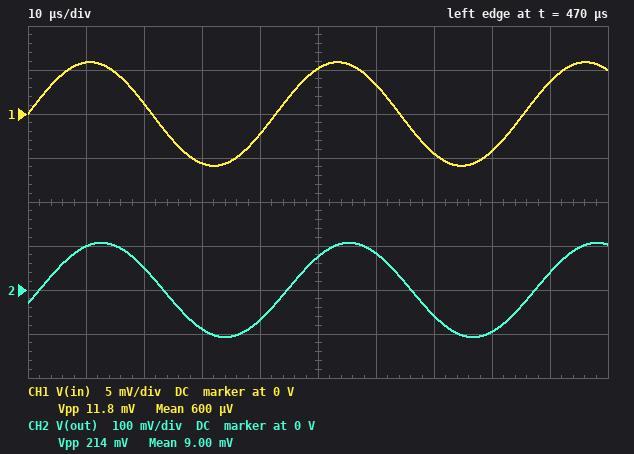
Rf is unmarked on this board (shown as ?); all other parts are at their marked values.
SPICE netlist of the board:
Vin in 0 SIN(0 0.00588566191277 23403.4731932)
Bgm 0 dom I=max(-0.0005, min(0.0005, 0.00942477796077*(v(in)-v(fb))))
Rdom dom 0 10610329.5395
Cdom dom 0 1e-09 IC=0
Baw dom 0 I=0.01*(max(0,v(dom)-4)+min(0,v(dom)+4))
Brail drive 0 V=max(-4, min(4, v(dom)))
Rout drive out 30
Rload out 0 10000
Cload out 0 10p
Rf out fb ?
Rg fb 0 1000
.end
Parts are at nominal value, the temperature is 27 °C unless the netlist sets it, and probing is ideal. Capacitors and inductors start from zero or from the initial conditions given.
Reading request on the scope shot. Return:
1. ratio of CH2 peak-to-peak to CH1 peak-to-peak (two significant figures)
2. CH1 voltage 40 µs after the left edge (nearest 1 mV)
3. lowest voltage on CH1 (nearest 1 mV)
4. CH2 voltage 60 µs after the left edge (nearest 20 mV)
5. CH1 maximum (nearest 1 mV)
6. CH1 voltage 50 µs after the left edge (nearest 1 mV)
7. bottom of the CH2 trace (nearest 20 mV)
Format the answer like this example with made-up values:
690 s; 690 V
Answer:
18; -2 mV; -6 mV; 80 mV; 6 mV; 5 mV; -100 mV
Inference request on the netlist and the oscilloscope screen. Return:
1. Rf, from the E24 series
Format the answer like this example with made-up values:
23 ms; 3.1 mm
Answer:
18 kΩ
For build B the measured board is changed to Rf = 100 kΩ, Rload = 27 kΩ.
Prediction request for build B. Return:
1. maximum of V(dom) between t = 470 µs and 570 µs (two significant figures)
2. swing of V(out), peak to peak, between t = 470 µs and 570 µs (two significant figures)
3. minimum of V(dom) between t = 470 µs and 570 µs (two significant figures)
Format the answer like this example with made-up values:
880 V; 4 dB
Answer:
320 mV; 640 mV; -320 mV
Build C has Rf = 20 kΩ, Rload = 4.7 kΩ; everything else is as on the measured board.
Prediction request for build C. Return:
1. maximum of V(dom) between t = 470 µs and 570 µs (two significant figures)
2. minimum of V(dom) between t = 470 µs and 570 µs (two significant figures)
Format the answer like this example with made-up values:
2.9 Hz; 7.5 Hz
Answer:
120 mV; -120 mV
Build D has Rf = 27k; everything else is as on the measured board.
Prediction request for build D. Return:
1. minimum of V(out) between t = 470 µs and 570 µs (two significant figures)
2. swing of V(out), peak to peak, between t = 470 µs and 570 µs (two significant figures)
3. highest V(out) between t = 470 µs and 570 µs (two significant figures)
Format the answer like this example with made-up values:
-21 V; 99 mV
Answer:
-150 mV; 300 mV; 150 mV
